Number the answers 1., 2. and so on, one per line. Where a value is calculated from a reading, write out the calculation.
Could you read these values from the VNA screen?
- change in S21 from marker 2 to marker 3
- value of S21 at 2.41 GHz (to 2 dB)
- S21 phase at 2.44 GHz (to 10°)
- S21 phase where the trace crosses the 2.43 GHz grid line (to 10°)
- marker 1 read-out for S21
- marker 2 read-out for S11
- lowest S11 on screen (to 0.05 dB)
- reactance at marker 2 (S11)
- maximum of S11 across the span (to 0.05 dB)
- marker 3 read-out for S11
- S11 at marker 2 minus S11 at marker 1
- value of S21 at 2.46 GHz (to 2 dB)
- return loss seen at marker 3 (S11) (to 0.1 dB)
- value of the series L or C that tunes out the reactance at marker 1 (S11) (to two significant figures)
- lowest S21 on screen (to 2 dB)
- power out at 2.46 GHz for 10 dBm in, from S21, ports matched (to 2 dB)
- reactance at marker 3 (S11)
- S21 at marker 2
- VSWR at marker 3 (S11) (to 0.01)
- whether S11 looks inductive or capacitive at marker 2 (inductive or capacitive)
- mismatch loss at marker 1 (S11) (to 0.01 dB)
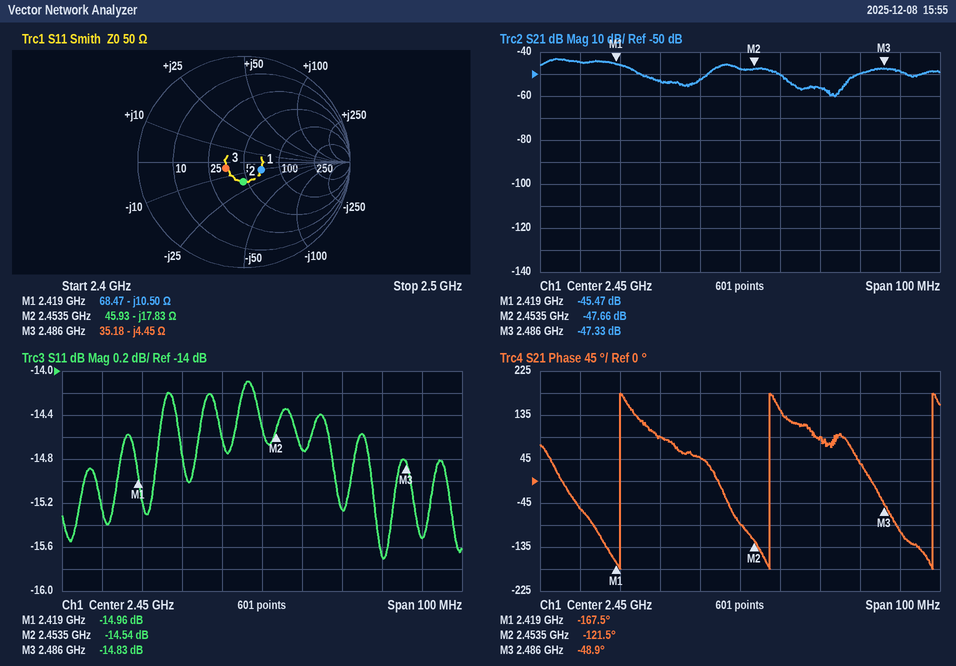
1. -47.33 − (-47.66) = 0.33 dB
2. -44 dB
3. 50°
4. 90°
5. -45.47 dB
6. -14.54 dB
7. -15.70 dB
8. -17.83 Ω
9. -14.10 dB
10. -14.83 dB
11. -14.54 − (-14.96) = 0.42 dB
12. -50 dB
13. 14.8 dB
14. L = 10.5 Ω/(2π × 2.419 GHz) ≈ 691 pH, so 690 pH to two significant figures
15. -60 dB
16. 10 dBm + (-50 dB) = -40 dBm
17. -4.45 Ω
18. -47.66 dB
19. (1 + 0.1813)/(1 − 0.1813) ≈ 1.44
20. capacitive
21. −10 log10(1 − 10^(-14.96/10)) ≈ 0.14 dB
